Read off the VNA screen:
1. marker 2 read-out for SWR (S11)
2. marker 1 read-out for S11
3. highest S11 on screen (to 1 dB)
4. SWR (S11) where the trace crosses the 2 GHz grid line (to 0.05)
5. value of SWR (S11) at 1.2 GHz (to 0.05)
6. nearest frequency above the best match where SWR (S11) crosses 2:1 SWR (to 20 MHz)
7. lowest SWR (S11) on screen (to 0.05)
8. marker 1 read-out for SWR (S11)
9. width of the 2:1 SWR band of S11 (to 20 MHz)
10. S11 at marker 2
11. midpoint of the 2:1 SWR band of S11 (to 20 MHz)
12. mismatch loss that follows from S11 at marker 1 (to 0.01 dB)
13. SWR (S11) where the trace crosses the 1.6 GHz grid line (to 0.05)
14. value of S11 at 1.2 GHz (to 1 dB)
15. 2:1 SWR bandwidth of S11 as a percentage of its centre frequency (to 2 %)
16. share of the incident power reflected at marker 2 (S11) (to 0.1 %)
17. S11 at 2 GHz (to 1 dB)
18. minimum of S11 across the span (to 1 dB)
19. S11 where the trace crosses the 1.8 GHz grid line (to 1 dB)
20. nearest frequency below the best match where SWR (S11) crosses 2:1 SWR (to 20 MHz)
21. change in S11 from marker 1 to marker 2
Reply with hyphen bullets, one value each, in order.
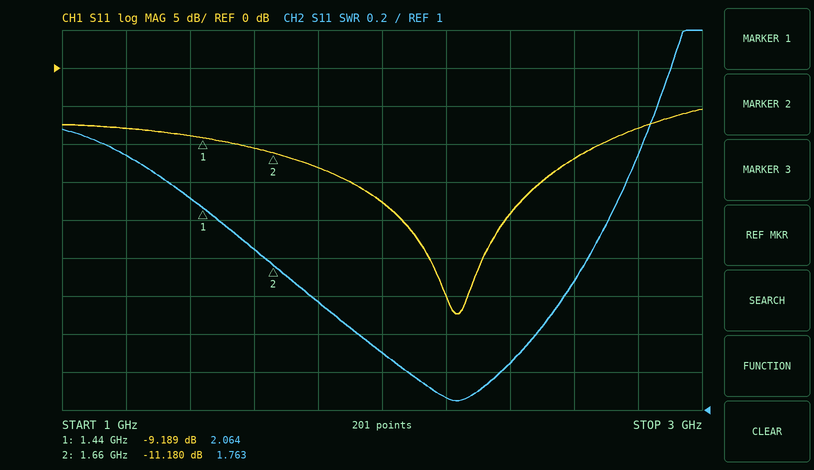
- 1.763
- -9.189 dB
- -5 dB
- 1.30
- 2.35
- 2.70 GHz
- 1.05
- 2.064
- 1.22 GHz
- -11.180 dB
- 2.10 GHz
- 0.56 dB
- 1.85
- -8 dB
- 58 %
- 7.6 %
- -18 dB
- -32 dB
- -13 dB
- 1.48 GHz
- -1.991 dB
